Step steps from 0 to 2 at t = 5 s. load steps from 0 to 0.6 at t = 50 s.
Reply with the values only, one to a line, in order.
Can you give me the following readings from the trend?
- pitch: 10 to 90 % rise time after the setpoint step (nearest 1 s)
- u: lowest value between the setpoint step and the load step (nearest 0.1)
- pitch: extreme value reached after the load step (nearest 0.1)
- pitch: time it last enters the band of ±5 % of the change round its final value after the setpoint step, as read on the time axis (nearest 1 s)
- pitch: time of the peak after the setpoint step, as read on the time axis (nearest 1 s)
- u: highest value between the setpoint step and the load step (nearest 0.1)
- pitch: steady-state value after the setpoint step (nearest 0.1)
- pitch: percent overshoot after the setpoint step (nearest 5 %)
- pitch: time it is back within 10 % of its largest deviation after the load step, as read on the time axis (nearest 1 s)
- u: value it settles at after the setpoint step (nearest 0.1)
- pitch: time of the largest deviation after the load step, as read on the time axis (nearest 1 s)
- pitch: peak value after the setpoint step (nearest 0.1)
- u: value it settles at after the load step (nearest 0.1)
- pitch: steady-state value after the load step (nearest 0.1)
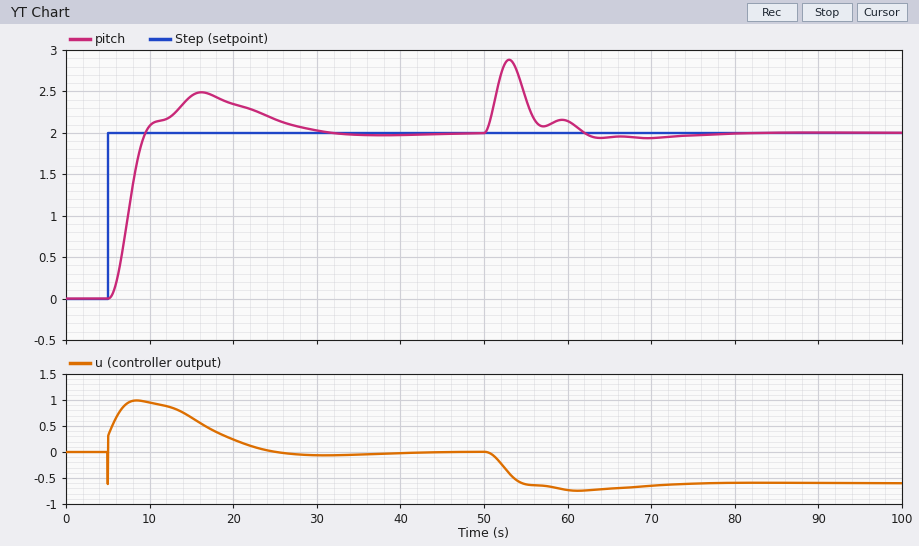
3 s
-0.6
2.9
27 s
16 s
1.0
2.0
25 %
61 s
0.0
53 s
2.5
-0.6
2.0
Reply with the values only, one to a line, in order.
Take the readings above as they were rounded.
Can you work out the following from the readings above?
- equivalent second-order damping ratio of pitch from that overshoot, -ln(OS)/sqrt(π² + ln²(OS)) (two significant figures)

0.40
